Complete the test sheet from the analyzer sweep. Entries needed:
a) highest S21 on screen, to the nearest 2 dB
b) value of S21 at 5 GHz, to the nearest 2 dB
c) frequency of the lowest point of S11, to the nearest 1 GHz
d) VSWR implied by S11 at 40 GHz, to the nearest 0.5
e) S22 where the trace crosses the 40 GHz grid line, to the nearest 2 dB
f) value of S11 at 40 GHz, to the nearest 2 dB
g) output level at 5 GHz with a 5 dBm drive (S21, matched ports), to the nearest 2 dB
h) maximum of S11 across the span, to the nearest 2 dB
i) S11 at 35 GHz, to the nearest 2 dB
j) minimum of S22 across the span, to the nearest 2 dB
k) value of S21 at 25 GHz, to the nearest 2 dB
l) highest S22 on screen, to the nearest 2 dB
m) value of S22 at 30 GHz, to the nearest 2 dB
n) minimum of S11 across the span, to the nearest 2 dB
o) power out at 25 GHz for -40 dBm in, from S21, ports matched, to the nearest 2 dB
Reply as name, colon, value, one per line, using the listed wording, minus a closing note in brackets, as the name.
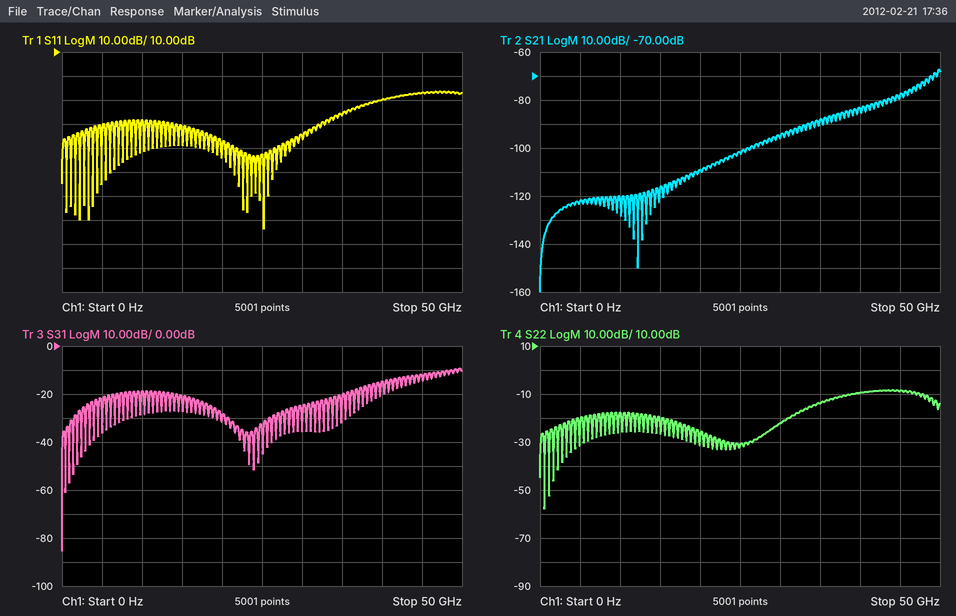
highest S21 on screen, to the nearest 2 dB: -68 dB
value of S21 at 5 GHz, to the nearest 2 dB: -122 dB
frequency of the lowest point of S11, to the nearest 1 GHz: 25 GHz
VSWR implied by S11 at 40 GHz, to the nearest 0.5: 2.0
S22 where the trace crosses the 40 GHz grid line, to the nearest 2 dB: -10 dB
value of S11 at 40 GHz, to the nearest 2 dB: -10 dB
output level at 5 GHz with a 5 dBm drive (S21, matched ports), to the nearest 2 dB: -118 dBm
maximum of S11 across the span, to the nearest 2 dB: -6 dB
S11 at 35 GHz, to the nearest 2 dB: -16 dB
minimum of S22 across the span, to the nearest 2 dB: -58 dB
value of S21 at 25 GHz, to the nearest 2 dB: -102 dB
highest S22 on screen, to the nearest 2 dB: -8 dB
value of S22 at 30 GHz, to the nearest 2 dB: -22 dB
minimum of S11 across the span, to the nearest 2 dB: -64 dB
power out at 25 GHz for -40 dBm in, from S21, ports matched, to the nearest 2 dB: -142 dBm
